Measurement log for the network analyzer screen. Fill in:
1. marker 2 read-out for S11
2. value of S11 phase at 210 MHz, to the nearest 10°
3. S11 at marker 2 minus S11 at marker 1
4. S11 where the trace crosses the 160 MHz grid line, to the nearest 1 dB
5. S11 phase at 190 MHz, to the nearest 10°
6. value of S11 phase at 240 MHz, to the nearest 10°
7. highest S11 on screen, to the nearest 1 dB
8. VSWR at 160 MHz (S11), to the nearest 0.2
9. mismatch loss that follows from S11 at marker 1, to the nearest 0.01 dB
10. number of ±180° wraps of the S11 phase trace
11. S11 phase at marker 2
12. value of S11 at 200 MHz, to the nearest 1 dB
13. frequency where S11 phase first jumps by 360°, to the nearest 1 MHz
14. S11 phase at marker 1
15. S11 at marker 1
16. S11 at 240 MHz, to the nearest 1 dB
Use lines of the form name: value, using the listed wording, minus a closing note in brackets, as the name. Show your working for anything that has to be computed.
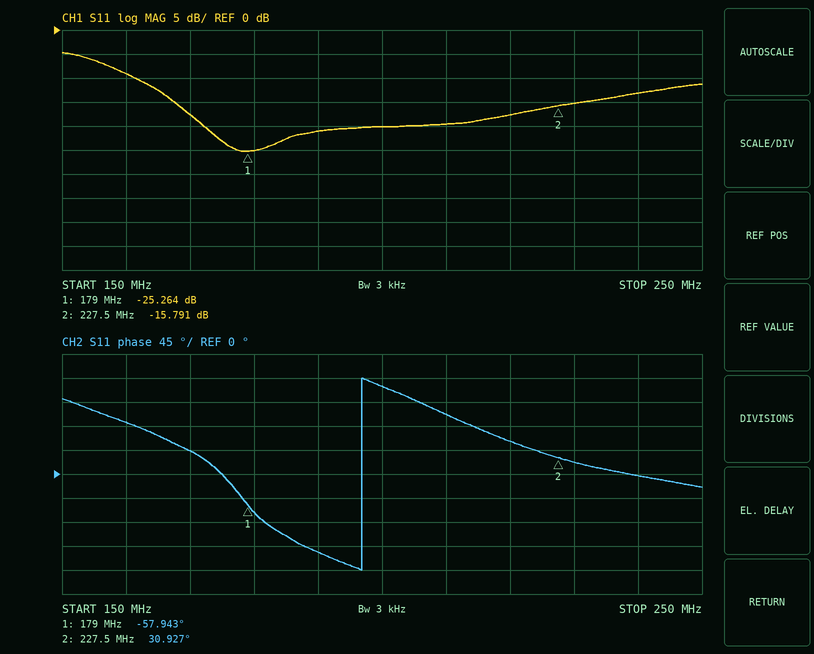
marker 2 read-out for S11: -15.791 dB
value of S11 phase at 210 MHz, to the nearest 10°: 110°
S11 at marker 2 minus S11 at marker 1: -15.791 − (-25.264) = 9.473 dB
S11 where the trace crosses the 160 MHz grid line, to the nearest 1 dB: -9 dB
S11 phase at 190 MHz, to the nearest 10°: -150°
value of S11 phase at 240 MHz, to the nearest 10°: 0°
highest S11 on screen, to the nearest 1 dB: -5 dB
VSWR at 160 MHz (S11), to the nearest 0.2: |Γ| = 10^(-9/20) = 0.3548; VSWR = (1 + 0.3548)/(1 − 0.3548) ≈ 2.10, so 2.0 to the nearest 0.2
mismatch loss that follows from S11 at marker 1, to the nearest 0.01 dB: −10 log10(1 − 10^(-25.264/10)) ≈ 0.01 dB
number of ±180° wraps of the S11 phase trace: 1
S11 phase at marker 2: 30.927°
value of S11 at 200 MHz, to the nearest 1 dB: -20 dB
frequency where S11 phase first jumps by 360°, to the nearest 1 MHz: 197 MHz
S11 phase at marker 1: -57.943°
S11 at marker 1: -25.264 dB
S11 at 240 MHz, to the nearest 1 dB: -13 dB
